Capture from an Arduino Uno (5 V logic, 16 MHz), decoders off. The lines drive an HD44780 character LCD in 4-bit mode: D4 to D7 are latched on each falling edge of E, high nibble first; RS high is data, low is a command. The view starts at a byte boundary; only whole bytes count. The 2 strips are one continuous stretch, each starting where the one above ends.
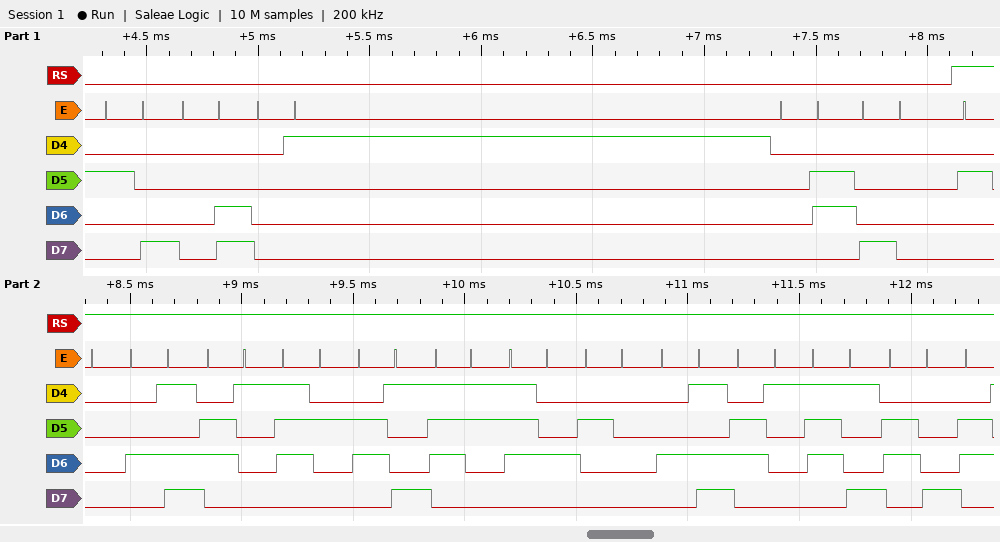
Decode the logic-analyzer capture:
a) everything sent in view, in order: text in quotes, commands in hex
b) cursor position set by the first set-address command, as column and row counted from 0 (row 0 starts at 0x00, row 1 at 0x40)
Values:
0x28 0x0C 0x01 0x06 0x80 " Marist Mayh"
column 0, row 0
